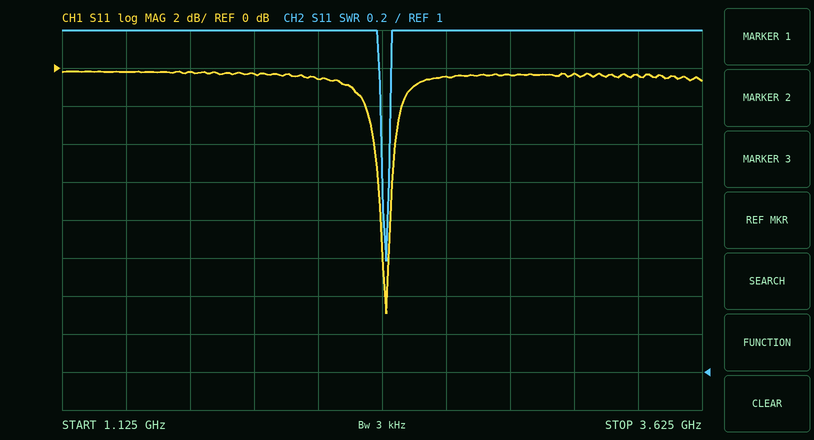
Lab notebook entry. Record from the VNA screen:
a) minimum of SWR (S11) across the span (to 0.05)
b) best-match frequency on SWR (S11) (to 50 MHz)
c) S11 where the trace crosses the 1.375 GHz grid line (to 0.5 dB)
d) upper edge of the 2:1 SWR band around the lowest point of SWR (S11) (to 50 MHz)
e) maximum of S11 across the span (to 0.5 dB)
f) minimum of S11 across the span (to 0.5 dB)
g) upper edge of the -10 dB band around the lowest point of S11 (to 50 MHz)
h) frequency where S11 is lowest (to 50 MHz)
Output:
1.60
2.40 GHz
0.0 dB
2.40 GHz
0.0 dB
-13.0 dB
2.40 GHz
2.40 GHz
